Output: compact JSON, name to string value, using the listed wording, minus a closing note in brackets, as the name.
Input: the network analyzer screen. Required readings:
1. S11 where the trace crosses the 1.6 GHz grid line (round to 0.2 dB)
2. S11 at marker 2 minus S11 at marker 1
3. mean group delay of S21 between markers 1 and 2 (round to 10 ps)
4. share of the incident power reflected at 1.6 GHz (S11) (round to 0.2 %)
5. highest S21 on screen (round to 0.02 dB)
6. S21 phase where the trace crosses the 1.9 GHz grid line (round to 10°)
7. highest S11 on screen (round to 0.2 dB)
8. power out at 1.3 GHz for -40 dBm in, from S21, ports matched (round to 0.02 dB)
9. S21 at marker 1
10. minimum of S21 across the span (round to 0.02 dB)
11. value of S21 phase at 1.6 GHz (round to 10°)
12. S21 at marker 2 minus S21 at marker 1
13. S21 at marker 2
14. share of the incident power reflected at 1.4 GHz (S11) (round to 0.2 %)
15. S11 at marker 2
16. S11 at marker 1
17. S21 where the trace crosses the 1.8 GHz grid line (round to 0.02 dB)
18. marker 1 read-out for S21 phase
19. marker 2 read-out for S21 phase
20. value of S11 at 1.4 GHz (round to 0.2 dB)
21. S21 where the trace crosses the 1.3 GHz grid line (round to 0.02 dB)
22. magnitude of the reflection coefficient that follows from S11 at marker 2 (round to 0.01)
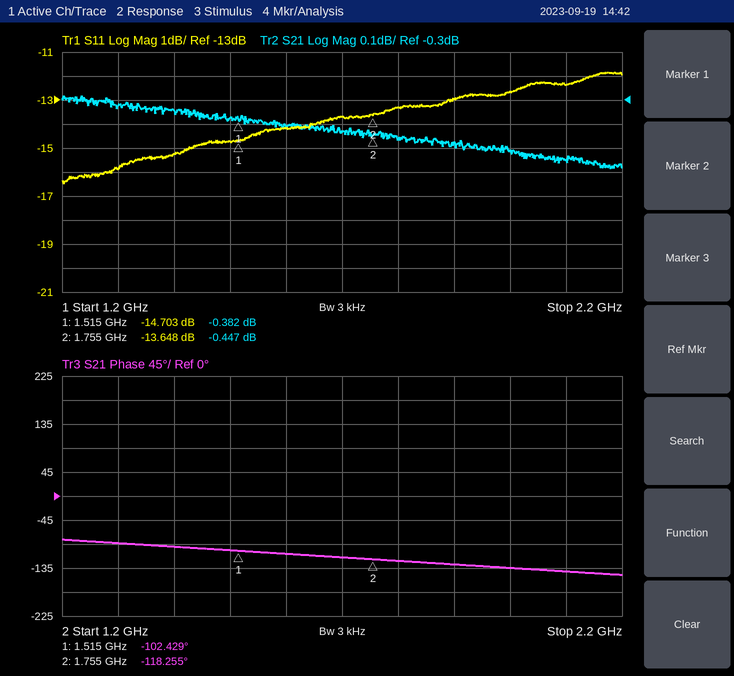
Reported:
{"S11 where the trace crosses the 1.6 GHz grid line": "-14.2 dB", "S11 at marker 2 minus S11 at marker 1": "1.055 dB", "mean group delay of S21 between markers 1 and 2": "180 ps", "share of the incident power reflected at 1.6 GHz (S11)": "3.8 %", "highest S21 on screen": "-0.28 dB", "S21 phase where the trace crosses the 1.9 GHz grid line": "-130°", "highest S11 on screen": "-11.8 dB", "power out at 1.3 GHz for -40 dBm in, from S21, ports matched": "-40.32 dBm", "S21 at marker 1": "-0.382 dB", "minimum of S21 across the span": "-0.58 dB", "value of S21 phase at 1.6 GHz": "-110°", "S21 at marker 2 minus S21 at marker 1": "-0.065 dB", "S21 at marker 2": "-0.447 dB", "share of the incident power reflected at 1.4 GHz (S11)": "3.0 %", "S11 at marker 2": "-13.648 dB", "S11 at marker 1": "-14.703 dB", "S21 where the trace crosses the 1.8 GHz grid line": "-0.46 dB", "marker 1 read-out for S21 phase": "-102.429°", "marker 2 read-out for S21 phase": "-118.255°", "value of S11 at 1.4 GHz": "-15.2 dB", "S21 where the trace crosses the 1.3 GHz grid line": "-0.32 dB", "magnitude of the reflection coefficient that follows from S11 at marker 2": "0.21"}
